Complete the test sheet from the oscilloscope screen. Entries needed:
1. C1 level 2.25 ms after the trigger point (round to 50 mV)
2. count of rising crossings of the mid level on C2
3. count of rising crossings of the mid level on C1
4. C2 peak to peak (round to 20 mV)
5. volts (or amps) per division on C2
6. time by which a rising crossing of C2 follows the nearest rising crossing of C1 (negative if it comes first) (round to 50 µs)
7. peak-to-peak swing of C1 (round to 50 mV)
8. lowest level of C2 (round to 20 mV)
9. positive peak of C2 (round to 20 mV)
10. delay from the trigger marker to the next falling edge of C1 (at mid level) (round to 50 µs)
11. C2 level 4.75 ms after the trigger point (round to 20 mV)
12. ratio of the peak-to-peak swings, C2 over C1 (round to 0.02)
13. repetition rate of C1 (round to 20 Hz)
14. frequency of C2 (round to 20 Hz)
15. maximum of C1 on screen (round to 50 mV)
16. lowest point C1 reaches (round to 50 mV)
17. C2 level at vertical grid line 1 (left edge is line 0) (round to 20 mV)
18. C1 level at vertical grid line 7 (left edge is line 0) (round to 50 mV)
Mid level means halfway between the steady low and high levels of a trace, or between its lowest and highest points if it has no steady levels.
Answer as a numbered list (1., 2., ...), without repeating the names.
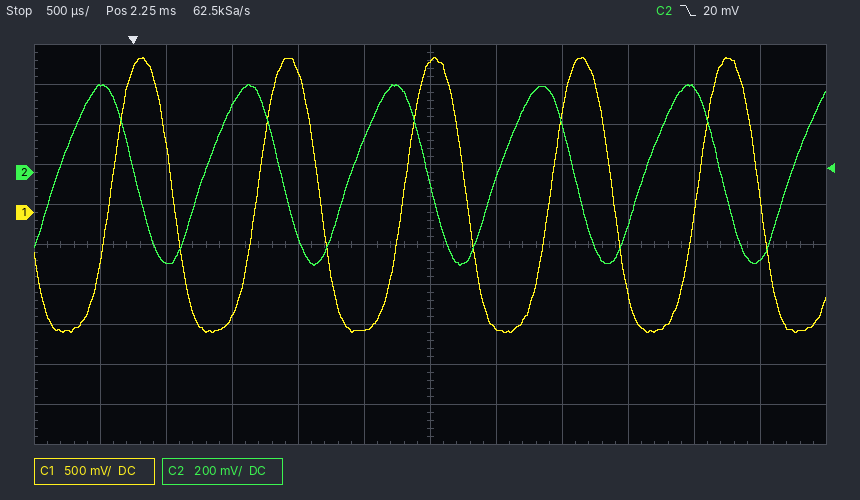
1. 1.90 V
2. 6
3. 5
4. 900 mV
5. 200 mV
6. -400 µs
7. 3.45 V
8. -460 mV
9. 440 mV
10. 300 µs
11. -440 mV
12. 0.26
13. 900 Hz
14. 900 Hz
15. 1.95 V
16. -1.50 V
17. 440 mV
18. -1.45 V
